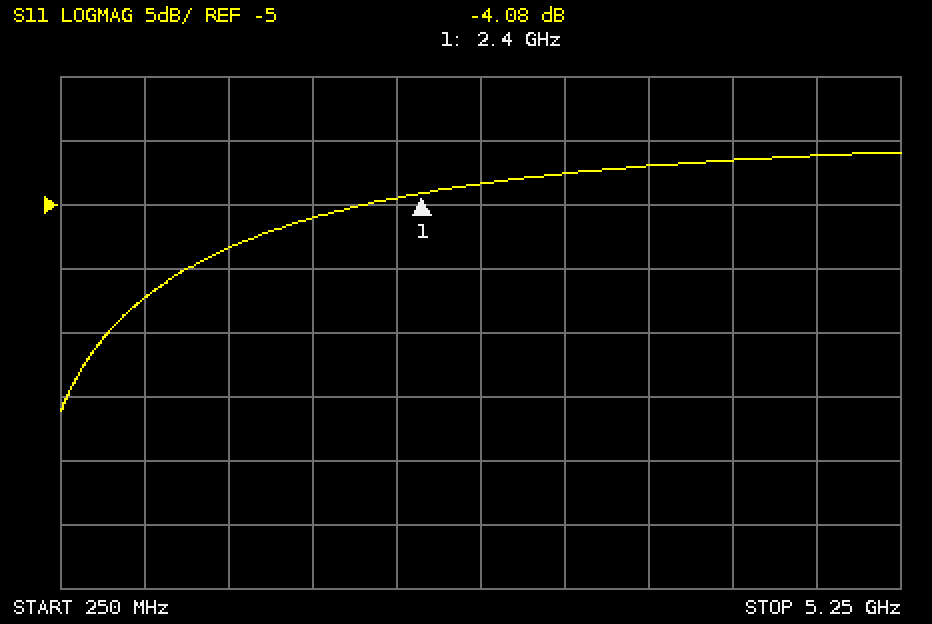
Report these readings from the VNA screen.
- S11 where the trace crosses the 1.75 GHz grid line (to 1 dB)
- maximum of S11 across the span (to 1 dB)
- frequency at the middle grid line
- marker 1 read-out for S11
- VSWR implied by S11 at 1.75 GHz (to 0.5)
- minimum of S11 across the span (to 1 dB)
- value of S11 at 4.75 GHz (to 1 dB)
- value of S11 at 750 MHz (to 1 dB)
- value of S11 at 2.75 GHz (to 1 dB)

-6 dB
-1 dB
2.75 GHz
-4.08 dB
3.0
-21 dB
-1 dB
-12 dB
-3 dB
